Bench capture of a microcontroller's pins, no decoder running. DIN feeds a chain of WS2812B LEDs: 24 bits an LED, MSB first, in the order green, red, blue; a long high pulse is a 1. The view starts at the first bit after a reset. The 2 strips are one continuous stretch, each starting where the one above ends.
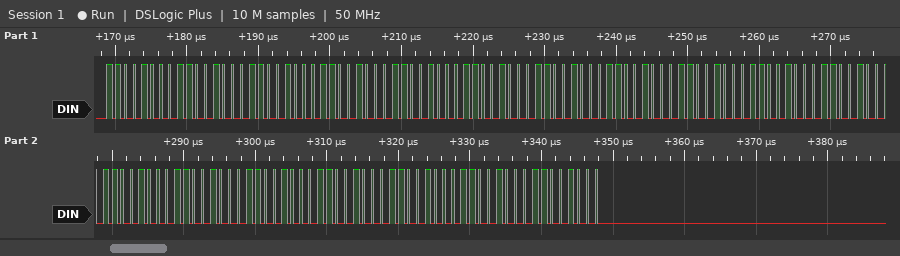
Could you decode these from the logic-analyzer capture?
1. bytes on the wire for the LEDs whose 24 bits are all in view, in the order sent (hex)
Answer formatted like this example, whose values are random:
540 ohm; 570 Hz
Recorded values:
C8 C8 C8 C8 C8 C8 C8 C8 C8 C8 C8 C8 C8 C8 C8 C8 C8 C8
